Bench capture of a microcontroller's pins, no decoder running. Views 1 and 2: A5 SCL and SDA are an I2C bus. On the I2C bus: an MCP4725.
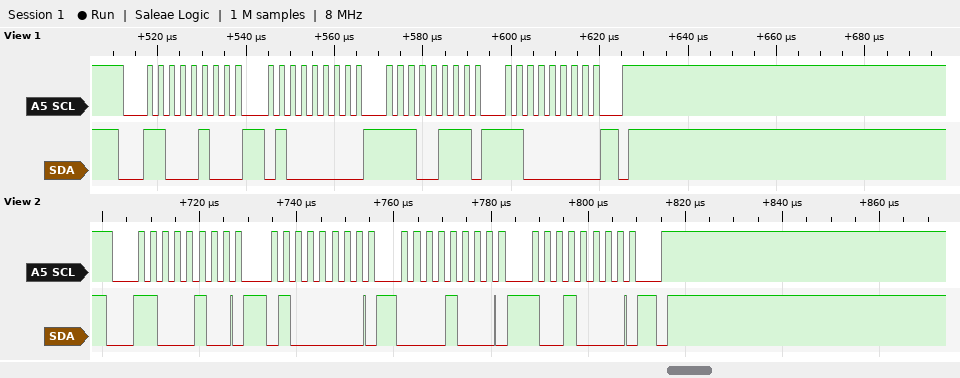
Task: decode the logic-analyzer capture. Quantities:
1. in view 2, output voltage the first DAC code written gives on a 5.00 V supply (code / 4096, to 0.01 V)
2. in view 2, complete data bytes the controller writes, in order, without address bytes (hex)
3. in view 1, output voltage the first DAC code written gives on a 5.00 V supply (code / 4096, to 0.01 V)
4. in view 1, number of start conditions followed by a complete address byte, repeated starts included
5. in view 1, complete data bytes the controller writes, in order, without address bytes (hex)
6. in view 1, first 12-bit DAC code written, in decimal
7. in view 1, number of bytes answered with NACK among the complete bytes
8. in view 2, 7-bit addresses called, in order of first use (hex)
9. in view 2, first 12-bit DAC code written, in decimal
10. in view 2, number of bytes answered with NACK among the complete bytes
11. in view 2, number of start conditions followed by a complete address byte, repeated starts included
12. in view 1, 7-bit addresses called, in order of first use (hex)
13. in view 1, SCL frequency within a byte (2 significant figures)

0.17 V
40 08 90
4.53 V
1
40 E7 C0
3708
0
0x62
137
0
1
0x62
400 kHz
